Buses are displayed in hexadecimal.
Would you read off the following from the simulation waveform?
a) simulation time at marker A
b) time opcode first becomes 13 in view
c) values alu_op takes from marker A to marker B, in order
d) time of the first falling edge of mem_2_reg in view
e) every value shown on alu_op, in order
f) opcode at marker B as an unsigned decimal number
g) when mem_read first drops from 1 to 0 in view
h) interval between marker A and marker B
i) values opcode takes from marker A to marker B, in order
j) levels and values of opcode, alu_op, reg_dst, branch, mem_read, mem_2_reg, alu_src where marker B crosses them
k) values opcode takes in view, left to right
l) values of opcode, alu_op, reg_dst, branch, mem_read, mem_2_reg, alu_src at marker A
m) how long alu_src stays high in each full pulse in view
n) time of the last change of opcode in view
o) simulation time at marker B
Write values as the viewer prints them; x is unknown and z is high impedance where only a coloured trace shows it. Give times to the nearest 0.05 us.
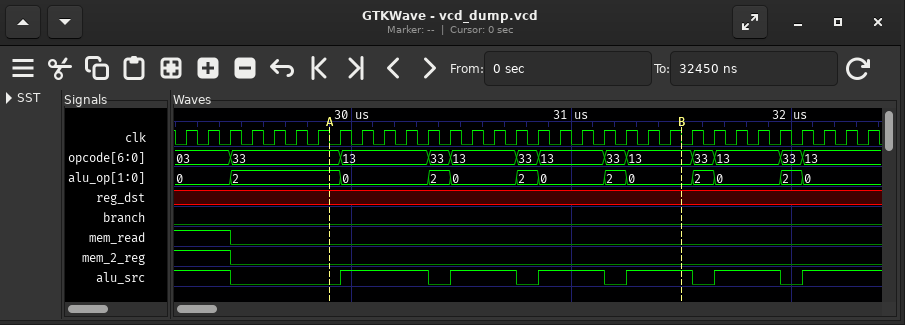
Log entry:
29.9 us
29.95 us
2, 0, 2, 0, 2, 0, 2, 0
29.45 us
0, 2, 0, 2, 0, 2, 0, 2, 0, 2, 0, 2, 0
19
29.45 us
1.6 us
33, 13, 33, 13, 33, 13, 33, 13
opcode=13, alu_op=0, reg_dst=x, branch=0, mem_read=0, mem_2_reg=0, alu_src=1
03, 33, 13, 33, 13, 33, 13, 33, 13, 33, 13, 33, 13
opcode=33, alu_op=2, reg_dst=x, branch=0, mem_read=0, mem_2_reg=0, alu_src=0
0.4 us, 0.3 us, 0.3 us, 0.3 us, 0.3 us
32.05 us
31.5 us
